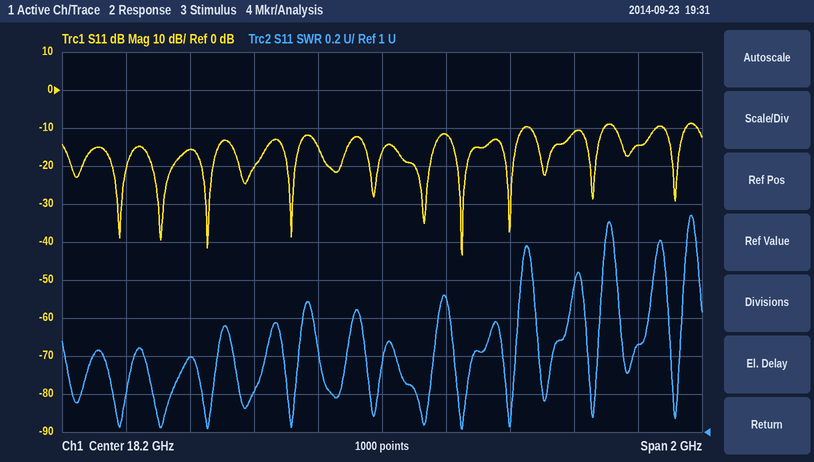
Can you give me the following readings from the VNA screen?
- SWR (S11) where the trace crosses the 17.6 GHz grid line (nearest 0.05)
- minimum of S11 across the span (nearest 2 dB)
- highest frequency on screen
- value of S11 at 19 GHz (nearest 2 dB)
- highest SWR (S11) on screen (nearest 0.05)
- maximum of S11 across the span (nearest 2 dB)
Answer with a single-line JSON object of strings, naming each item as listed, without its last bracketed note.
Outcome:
{"SWR (S11) where the trace crosses the 17.6 GHz grid line": "1.40", "minimum of S11 across the span": "-44 dB", "highest frequency on screen": "19.2 GHz", "value of S11 at 19 GHz": "-14 dB", "highest SWR (S11) on screen": "2.15", "maximum of S11 across the span": "-8 dB"}
